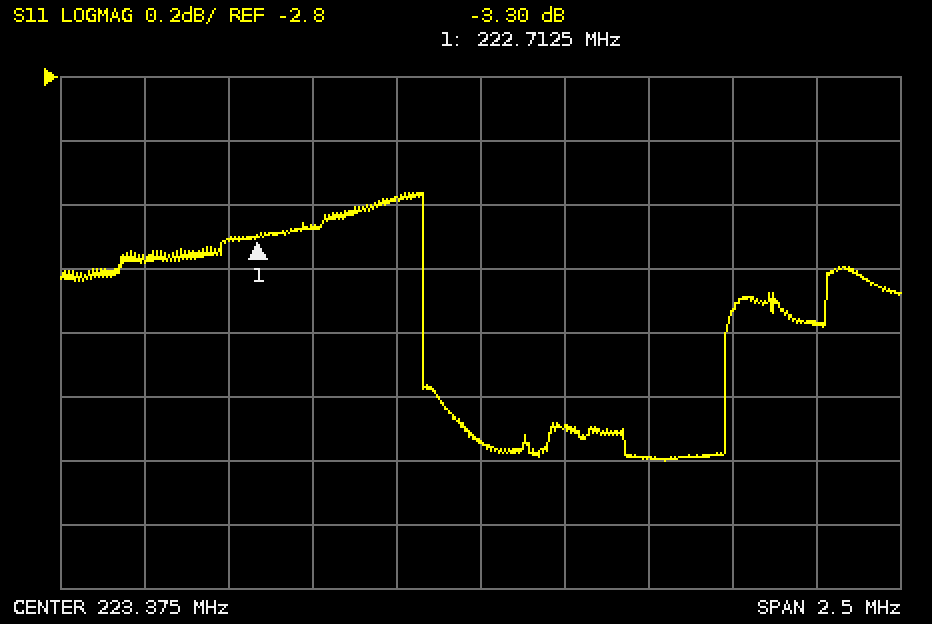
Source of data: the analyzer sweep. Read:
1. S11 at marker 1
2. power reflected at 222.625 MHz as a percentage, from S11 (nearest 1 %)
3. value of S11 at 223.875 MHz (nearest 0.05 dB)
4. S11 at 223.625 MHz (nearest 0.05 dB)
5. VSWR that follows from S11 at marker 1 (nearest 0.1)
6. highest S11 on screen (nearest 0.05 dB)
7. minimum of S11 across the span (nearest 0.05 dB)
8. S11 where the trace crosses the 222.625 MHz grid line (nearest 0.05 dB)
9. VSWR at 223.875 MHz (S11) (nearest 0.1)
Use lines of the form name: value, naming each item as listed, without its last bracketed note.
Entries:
S11 at marker 1: -3.30 dB
power reflected at 222.625 MHz as a percentage, from S11: 47 %
value of S11 at 223.875 MHz: -4.00 dB
S11 at 223.625 MHz: -3.90 dB
VSWR that follows from S11 at marker 1: 5.3
highest S11 on screen: -3.15 dB
minimum of S11 across the span: -4.00 dB
S11 where the trace crosses the 222.625 MHz grid line: -3.30 dB
VSWR at 223.875 MHz (S11): 4.4
